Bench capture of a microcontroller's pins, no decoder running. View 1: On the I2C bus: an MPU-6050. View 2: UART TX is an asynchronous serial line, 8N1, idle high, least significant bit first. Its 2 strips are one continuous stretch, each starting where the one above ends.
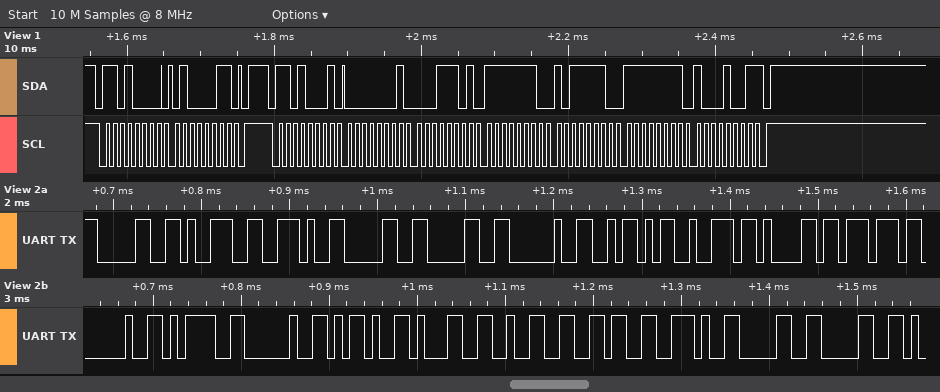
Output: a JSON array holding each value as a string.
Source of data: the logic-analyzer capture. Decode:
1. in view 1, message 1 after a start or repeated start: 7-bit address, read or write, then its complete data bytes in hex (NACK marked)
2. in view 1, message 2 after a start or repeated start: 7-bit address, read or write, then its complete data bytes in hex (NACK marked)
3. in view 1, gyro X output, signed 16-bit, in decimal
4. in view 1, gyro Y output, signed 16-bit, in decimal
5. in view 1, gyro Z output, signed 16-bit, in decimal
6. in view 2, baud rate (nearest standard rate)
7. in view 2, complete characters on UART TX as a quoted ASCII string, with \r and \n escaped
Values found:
["0x68 write: 43", "0x68 read: 01 1D FE BE FF 89 NACK", "285", "-322", "-119", "115200 baud", "\"09.00 Zraw = -126.00\""]
